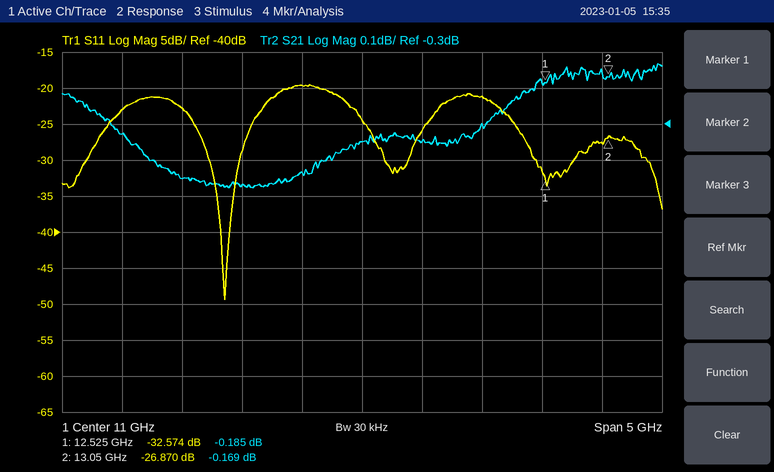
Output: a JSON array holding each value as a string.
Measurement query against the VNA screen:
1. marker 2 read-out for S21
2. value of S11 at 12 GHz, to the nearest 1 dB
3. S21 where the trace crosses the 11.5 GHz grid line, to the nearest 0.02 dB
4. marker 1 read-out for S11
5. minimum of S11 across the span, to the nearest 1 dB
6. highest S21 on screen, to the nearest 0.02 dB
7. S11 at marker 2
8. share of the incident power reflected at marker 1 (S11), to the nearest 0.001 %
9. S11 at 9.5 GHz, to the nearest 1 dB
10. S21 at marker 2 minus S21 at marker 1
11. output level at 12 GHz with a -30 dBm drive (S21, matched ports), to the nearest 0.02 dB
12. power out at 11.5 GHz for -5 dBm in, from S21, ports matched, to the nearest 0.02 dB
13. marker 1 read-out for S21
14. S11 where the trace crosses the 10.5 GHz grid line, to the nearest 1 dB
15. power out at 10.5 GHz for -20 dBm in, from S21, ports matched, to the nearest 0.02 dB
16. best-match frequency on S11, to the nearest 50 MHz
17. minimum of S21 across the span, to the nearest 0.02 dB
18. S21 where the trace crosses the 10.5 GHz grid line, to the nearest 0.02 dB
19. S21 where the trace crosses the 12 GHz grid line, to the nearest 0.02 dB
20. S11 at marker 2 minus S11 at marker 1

["-0.169 dB", "-21 dB", "-0.34 dB", "-32.574 dB", "-49 dB", "-0.14 dB", "-26.870 dB", "0.055 %", "-23 dB", "0.016 dB", "-30.30 dBm", "-5.34 dBm", "-0.185 dB", "-20 dB", "-20.44 dBm", "9.85 GHz", "-0.48 dB", "-0.44 dB", "-0.30 dB", "5.704 dB"]
